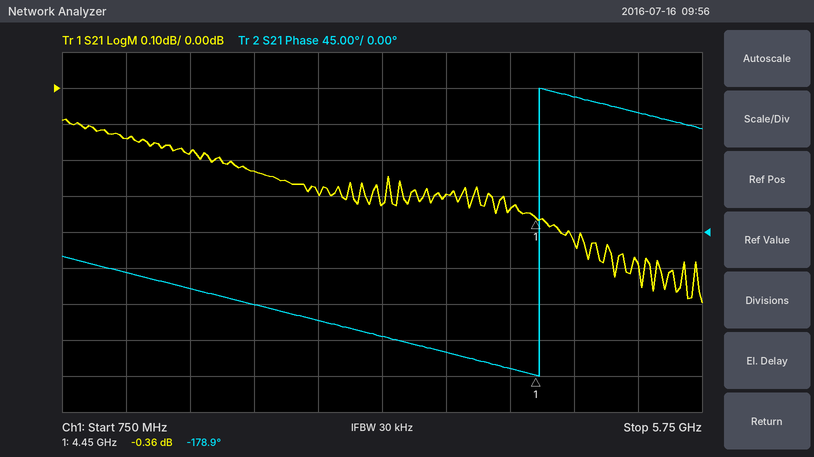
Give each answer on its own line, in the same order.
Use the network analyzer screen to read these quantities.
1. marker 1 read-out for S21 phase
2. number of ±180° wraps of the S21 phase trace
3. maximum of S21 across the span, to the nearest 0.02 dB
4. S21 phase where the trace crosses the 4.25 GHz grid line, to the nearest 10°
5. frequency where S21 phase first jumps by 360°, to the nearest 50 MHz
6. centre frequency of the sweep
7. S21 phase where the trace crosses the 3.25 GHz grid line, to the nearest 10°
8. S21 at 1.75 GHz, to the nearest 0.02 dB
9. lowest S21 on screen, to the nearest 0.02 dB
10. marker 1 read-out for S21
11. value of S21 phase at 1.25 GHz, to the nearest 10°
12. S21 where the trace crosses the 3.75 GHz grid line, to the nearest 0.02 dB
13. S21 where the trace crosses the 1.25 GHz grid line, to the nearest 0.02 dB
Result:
-178.9°
1
-0.08 dB
-170°
4.50 GHz
3.25 GHz
-130°
-0.18 dB
-0.60 dB
-0.36 dB
-50°
-0.30 dB
-0.14 dB
